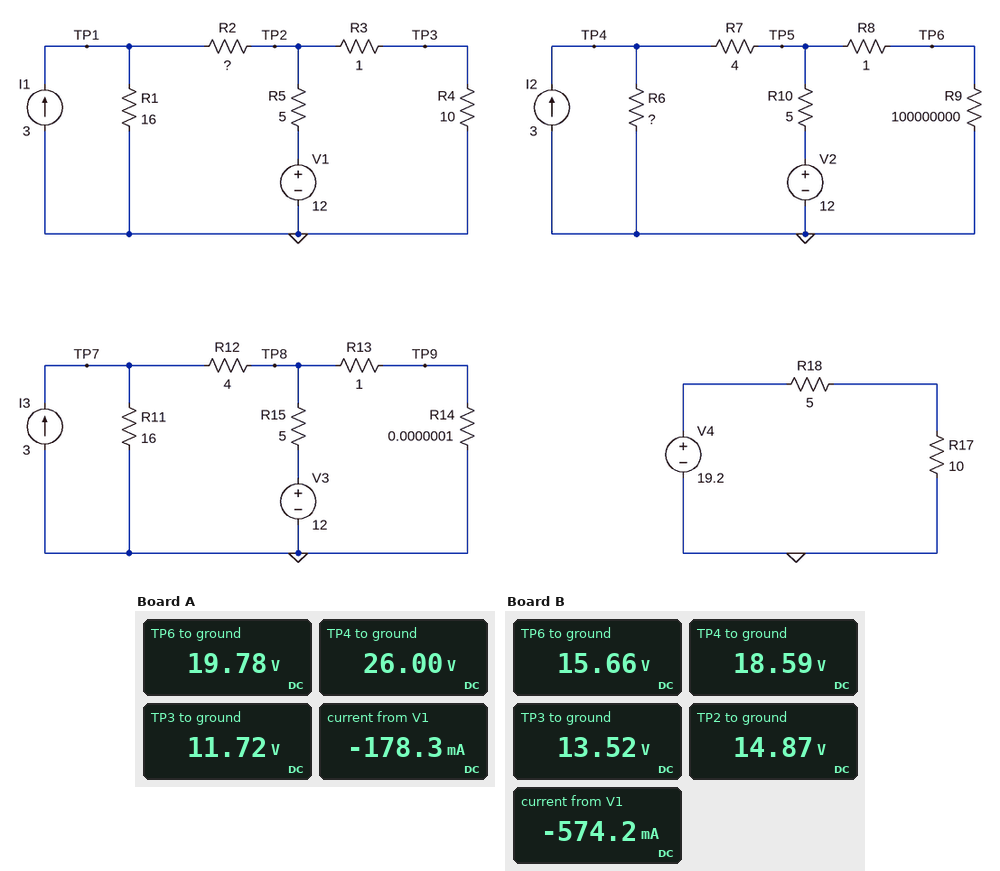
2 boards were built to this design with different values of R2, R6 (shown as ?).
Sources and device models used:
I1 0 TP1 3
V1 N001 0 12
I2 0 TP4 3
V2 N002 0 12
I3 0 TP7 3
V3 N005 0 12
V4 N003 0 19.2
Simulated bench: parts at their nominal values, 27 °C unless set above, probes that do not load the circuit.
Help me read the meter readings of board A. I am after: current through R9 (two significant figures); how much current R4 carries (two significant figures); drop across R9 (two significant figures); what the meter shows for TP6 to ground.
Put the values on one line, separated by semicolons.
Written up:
200 nA; 1.2 A; 20 V; 19.78 V
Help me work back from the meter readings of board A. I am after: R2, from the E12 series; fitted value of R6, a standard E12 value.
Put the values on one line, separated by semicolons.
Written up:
10 Ω; 18 Ω
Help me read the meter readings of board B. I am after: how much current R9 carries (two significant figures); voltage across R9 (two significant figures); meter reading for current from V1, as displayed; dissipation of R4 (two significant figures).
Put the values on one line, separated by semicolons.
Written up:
160 nA; 16 V; -574.2 mA; 18 W
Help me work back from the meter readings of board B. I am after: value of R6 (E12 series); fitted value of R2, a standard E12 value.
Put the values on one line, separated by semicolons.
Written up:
8.2 Ω; 1.2 Ω
